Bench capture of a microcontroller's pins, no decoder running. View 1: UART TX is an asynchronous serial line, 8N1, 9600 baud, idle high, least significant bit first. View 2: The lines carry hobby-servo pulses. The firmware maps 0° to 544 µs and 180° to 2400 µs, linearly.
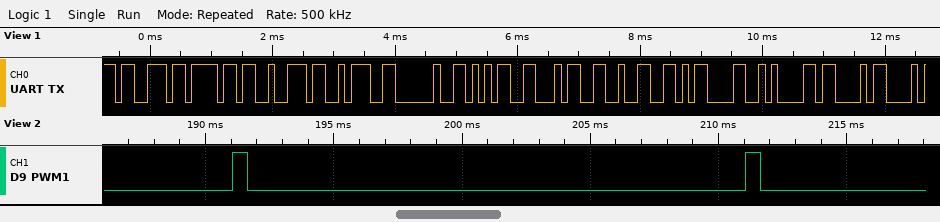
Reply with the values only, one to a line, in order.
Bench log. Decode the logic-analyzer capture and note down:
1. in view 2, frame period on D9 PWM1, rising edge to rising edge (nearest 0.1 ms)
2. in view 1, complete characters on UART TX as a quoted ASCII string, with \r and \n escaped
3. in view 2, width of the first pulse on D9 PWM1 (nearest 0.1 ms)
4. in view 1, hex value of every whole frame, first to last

20.0 ms
"sor: 542\r\nC"
0.6 ms
0x73 0x6F 0x72 0x3A 0x20 0x35 0x34 0x32 0x0D 0x0A 0x43
